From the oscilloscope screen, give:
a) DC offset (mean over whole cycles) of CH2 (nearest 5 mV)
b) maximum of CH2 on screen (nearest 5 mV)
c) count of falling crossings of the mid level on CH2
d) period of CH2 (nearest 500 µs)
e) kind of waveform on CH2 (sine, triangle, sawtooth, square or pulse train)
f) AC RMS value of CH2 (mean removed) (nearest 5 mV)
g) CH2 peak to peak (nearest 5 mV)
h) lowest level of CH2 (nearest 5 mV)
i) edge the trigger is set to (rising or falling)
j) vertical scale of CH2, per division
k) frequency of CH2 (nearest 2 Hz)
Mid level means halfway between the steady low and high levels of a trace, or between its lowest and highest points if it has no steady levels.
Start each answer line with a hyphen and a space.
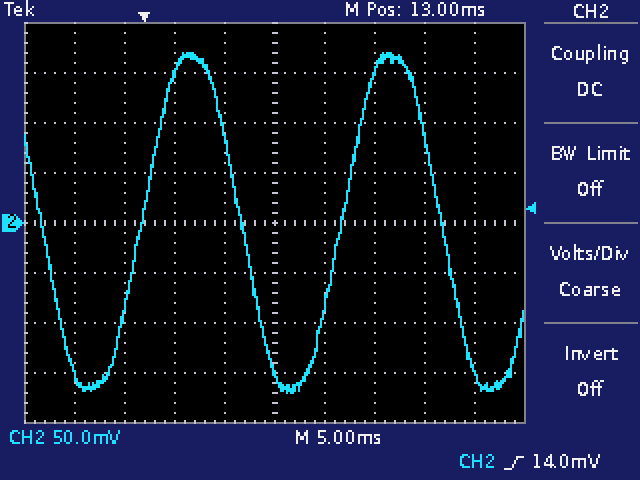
- 0 mV
- 170 mV
- 3
- 20.0 ms
- sine
- 120 mV
- 340 mV
- -170 mV
- rising
- 50 mV
- 50 Hz
